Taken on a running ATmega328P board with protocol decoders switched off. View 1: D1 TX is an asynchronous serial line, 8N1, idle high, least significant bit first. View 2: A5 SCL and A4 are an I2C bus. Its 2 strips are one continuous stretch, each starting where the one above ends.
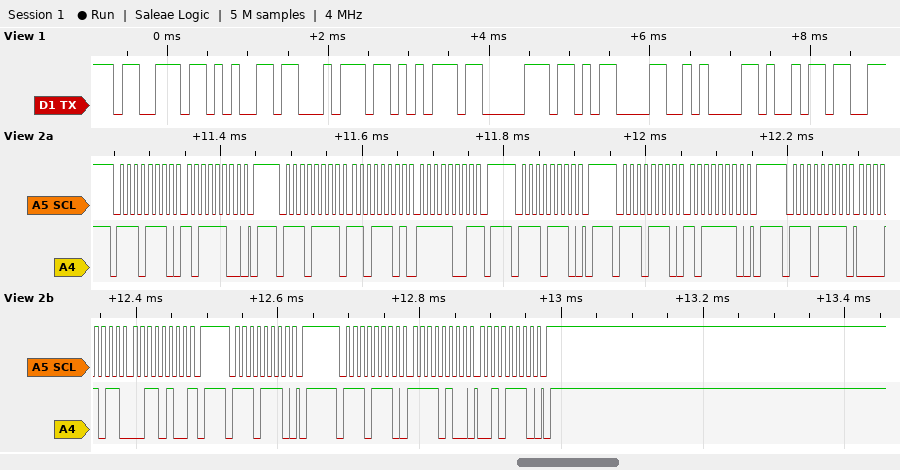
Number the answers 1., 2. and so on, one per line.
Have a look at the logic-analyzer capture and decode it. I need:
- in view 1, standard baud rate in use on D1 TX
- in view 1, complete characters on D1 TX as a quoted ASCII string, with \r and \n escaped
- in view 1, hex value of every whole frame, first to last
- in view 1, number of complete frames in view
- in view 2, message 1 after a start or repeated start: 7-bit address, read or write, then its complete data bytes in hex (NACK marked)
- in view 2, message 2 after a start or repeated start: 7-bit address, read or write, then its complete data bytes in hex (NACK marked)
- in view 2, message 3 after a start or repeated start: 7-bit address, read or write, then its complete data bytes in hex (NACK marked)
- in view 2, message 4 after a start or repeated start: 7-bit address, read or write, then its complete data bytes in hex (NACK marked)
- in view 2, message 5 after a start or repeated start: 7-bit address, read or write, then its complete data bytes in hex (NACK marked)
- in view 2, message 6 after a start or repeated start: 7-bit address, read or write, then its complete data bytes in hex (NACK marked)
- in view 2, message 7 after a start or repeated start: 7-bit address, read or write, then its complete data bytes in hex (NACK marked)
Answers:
1. 9600 baud
2. "setup\r\ni"
3. 73 65 74 75 70 0D 0A 69
4. 8
5. 0x77 write: BC
6. 0x77 read: DD F9 NACK
7. 0x77 write
8. 0x77 write: BE
9. 0x77 read: 0B 34 NACK
10. 0x77 write
11. 0x77 write: F4 2E
